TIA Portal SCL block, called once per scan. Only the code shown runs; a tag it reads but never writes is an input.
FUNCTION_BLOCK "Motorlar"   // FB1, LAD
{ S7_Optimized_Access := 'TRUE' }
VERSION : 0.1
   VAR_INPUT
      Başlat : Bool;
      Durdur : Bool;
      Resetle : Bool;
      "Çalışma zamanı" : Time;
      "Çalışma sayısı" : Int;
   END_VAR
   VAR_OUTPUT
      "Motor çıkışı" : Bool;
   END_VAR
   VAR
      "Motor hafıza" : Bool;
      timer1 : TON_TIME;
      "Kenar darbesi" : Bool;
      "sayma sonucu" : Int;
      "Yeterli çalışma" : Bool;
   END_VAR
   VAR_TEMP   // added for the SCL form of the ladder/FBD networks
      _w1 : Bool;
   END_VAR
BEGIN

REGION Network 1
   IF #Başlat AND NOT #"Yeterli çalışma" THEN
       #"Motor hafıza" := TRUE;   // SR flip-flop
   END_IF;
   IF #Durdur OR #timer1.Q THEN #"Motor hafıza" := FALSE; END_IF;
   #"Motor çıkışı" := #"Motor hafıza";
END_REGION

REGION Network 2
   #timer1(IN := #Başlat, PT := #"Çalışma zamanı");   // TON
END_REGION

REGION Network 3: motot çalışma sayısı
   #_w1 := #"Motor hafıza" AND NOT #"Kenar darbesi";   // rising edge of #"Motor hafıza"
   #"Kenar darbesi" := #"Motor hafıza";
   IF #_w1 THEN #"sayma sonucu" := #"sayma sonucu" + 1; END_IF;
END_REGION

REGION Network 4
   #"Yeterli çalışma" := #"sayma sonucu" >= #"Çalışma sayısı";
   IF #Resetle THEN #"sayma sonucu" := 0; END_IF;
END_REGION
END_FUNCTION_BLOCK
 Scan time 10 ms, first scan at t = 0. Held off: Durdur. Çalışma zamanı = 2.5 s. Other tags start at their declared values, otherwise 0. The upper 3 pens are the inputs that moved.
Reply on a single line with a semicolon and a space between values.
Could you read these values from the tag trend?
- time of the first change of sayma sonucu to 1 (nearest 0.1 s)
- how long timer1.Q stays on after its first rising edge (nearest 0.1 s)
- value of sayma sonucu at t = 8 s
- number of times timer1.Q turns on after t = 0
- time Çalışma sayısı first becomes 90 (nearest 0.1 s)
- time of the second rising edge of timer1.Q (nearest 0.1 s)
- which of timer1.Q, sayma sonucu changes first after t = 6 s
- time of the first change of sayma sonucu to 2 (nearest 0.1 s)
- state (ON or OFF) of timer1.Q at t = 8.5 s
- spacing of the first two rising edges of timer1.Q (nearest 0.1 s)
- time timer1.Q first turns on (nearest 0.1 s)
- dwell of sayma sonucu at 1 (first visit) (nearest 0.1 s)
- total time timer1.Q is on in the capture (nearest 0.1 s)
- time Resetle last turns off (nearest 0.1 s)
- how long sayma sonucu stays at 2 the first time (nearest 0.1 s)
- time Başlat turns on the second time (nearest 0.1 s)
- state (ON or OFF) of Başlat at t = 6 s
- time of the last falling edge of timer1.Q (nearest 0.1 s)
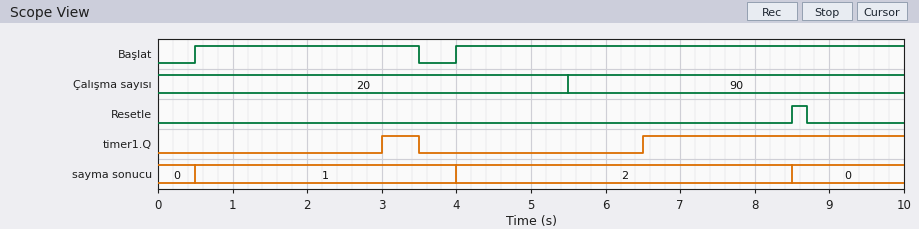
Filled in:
0.5 s; 0.5 s; 2; 2; 5.5 s; 6.5 s; timer1.Q; 4.0 s; ON; 3.5 s; 3.0 s; 3.5 s; 4.0 s; 8.7 s; 4.5 s; 4.0 s; ON; 3.5 s
